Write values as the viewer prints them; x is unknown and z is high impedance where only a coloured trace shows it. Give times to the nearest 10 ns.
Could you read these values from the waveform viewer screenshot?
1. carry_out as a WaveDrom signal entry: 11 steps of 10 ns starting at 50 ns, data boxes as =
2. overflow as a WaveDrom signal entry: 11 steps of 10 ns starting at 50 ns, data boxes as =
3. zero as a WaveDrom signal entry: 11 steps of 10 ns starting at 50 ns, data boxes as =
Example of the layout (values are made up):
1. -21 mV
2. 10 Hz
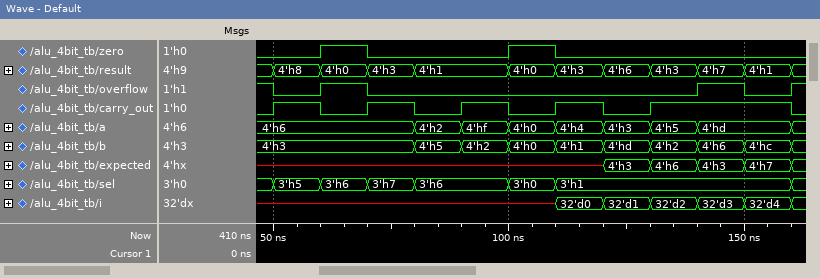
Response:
1. {name: 'carry_out', wave: '101010101..'}
2. {name: 'overflow', wave: '010......10'}
3. {name: 'zero', wave: '010..10....'}
